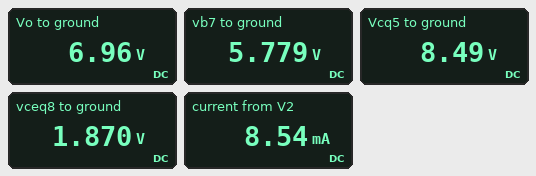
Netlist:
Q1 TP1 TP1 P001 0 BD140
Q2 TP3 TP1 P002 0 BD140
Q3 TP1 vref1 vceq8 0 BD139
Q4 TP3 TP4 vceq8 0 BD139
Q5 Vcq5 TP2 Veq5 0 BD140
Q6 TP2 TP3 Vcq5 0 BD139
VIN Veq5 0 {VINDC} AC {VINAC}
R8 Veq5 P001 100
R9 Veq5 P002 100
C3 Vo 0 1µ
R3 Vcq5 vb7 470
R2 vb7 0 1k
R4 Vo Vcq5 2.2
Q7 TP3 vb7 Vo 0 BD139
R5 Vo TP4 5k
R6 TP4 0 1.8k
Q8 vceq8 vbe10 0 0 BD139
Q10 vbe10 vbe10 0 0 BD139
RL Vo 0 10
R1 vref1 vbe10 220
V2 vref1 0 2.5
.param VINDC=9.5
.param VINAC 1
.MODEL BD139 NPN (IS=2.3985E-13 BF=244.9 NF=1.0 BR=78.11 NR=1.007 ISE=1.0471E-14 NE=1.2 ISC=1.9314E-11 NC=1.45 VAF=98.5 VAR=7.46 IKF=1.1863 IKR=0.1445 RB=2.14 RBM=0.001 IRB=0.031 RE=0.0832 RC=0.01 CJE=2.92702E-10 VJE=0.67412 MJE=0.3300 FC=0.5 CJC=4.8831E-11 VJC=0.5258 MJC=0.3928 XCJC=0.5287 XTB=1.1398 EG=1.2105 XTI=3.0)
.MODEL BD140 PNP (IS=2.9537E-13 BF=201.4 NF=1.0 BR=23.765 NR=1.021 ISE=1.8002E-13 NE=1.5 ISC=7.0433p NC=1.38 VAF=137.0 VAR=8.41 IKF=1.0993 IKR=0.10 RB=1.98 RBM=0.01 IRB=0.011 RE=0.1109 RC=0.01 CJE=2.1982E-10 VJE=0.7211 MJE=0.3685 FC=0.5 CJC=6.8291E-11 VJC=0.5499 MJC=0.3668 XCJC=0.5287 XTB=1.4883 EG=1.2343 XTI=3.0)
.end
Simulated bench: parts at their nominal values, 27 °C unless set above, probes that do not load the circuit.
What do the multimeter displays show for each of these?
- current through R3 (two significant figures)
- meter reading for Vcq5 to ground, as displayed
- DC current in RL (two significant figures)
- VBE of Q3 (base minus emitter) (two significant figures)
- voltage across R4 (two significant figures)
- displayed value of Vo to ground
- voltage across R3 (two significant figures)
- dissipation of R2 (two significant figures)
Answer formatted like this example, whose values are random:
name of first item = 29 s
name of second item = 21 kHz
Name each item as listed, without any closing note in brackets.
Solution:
current through R3 = 5.8 mA
meter reading for Vcq5 to ground, as displayed = 8.49 V
DC current in RL = 700 mA
VBE of Q3 (base minus emitter) = 630 mV
voltage across R4 = 1.5 V
displayed value of Vo to ground = 6.96 V
voltage across R3 = 2.7 V
dissipation of R2 = 33 mW
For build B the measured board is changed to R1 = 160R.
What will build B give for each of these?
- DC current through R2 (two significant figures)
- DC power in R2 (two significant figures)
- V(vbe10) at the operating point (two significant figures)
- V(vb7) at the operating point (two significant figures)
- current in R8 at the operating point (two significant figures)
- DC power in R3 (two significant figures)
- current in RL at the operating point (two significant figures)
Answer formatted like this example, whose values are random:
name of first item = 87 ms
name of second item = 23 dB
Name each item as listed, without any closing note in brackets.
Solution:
DC current through R2 = 5.7 mA
DC power in R2 = 32 mW
V(vbe10) at the operating point = 640 mV
V(vb7) at the operating point = 5.7 V
current in R8 at the operating point = 6.2 mA
DC power in R3 = 15 mW
current in RL at the operating point = 680 mA
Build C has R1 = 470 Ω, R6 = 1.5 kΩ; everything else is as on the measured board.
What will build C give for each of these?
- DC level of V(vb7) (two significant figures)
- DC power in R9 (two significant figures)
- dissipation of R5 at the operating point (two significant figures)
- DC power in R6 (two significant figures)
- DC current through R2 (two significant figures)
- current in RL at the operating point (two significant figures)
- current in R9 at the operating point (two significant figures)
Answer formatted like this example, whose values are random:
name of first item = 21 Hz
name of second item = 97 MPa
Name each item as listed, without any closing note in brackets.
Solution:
DC level of V(vb7) = 5.9 V
DC power in R9 = 440 µW
dissipation of R5 at the operating point = 5.9 mW
DC power in R6 = 1.8 mW
DC current through R2 = 5.9 mA
current in RL at the operating point = 710 mA
current in R9 at the operating point = 2.1 mA
